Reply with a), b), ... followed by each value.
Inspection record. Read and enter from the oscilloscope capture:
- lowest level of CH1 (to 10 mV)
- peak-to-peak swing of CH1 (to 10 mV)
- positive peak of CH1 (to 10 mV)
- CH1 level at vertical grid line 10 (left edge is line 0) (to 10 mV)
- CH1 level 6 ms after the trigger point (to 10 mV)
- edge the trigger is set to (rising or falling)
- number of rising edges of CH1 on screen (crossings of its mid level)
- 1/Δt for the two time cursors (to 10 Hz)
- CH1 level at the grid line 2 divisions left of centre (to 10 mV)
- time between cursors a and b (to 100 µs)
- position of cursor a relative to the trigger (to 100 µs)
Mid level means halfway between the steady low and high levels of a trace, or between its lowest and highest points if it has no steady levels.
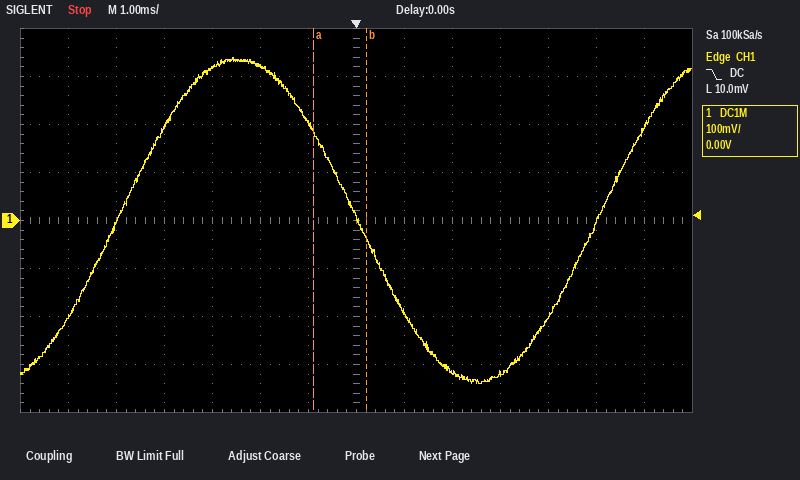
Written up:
a) -340 mV
b) 680 mV
c) 340 mV
d) -320 mV
e) 190 mV
f) falling
g) 2
h) 910 Hz
i) 320 mV
j) 1.1 ms
k) -900 µs
